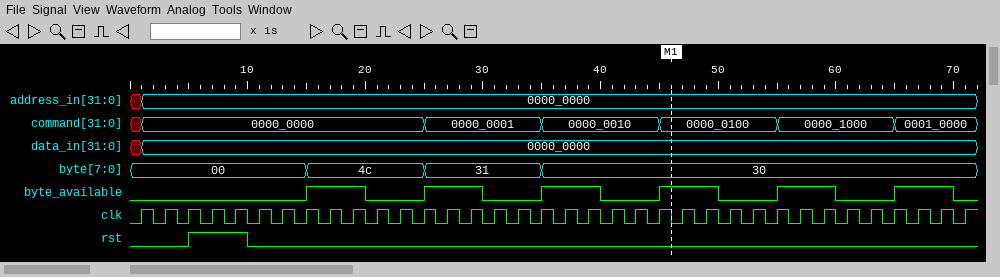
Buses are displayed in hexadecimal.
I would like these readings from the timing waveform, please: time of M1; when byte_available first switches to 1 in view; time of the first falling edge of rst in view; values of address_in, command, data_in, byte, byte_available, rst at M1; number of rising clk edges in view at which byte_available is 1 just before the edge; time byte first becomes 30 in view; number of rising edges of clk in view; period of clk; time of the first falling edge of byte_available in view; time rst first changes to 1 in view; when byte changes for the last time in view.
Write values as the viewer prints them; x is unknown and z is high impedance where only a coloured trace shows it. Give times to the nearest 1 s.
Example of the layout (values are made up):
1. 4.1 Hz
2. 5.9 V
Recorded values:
1. 46 s
2. 15 s
3. 10 s
4. address_in=0000_0000, command=0000_0100, data_in=0000_0000, byte=30, byte_available=1, rst=0
5. 12
6. 35 s
7. 36
8. 2 s
9. 20 s
10. 5 s
11. 35 s
